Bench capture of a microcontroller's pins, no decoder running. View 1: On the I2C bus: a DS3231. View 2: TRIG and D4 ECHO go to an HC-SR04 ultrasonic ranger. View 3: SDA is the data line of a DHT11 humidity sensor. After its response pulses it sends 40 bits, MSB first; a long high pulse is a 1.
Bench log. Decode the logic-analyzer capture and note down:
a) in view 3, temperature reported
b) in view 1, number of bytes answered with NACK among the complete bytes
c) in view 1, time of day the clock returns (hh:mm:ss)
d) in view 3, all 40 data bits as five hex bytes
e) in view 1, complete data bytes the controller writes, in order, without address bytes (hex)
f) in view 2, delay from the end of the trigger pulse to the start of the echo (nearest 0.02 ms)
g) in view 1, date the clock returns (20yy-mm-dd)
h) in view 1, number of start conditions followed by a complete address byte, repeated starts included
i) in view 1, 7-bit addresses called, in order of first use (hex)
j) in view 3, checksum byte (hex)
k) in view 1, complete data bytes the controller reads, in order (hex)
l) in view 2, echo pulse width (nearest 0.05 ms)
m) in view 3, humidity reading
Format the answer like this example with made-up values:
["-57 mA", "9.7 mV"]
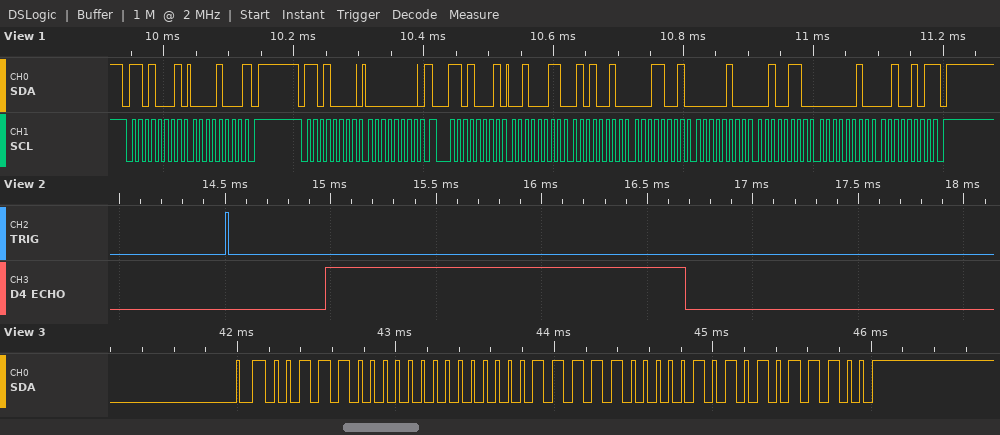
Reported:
["31.5 °C", "2", "19:52:23", "38 00 1F 05 5C", "00", "0.46 ms", "2025-02-26", "3", "0x68", "0x5C", "08 23 52 19 04 26 02 25", "1.70 ms", "56 %"]
